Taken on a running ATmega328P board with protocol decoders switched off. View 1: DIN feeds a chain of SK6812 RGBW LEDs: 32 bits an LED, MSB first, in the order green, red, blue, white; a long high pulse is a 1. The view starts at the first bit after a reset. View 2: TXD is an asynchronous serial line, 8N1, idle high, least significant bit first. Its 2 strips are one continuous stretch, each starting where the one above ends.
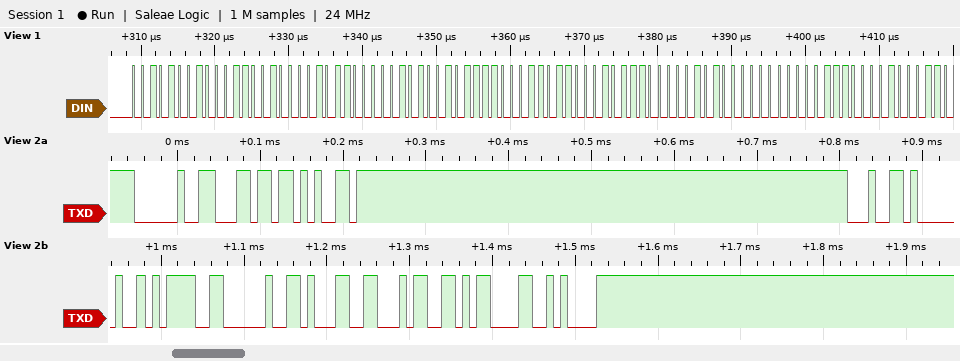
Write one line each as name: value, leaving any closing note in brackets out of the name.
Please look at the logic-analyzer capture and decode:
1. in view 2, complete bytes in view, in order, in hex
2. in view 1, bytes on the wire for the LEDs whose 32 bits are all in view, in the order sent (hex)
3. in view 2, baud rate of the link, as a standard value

in view 2, complete bytes in view, in order, in hex: 20 6C 65 64 20 3D 20 31 34 0D 0A
in view 1, bytes on the wire for the LEDs whose 32 bits are all in view, in the order sent: 29 19 0B 05 2F 1B 17 05
in view 2, baud rate of the link, as a standard value: 115200 baud
